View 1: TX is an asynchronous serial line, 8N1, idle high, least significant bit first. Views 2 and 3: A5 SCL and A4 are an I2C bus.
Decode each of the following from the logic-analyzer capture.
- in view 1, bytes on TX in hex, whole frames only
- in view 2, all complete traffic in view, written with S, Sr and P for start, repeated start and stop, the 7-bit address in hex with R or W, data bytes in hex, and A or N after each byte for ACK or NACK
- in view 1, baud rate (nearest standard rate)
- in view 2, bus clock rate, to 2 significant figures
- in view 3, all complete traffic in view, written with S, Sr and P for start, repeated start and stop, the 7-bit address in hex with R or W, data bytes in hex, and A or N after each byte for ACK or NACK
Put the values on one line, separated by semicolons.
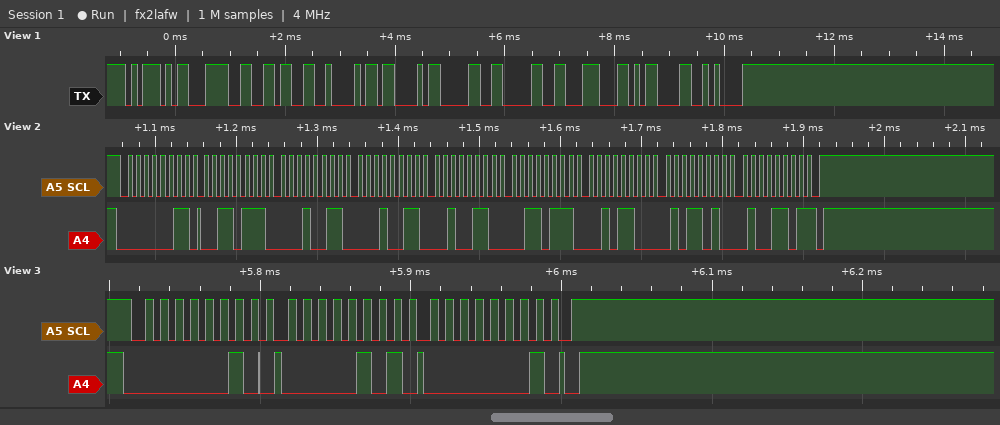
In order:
0x5D 0x3C 0x36 0x42 0x43 0x30 0x30 0x1C 0x0D 0x0A; S 01R A 37 A 13 A 13 A 26 A 37 A 2C A 5A A 4D N P; 9600 baud; 100 kHz; S 01W A 05 A 01 A P
